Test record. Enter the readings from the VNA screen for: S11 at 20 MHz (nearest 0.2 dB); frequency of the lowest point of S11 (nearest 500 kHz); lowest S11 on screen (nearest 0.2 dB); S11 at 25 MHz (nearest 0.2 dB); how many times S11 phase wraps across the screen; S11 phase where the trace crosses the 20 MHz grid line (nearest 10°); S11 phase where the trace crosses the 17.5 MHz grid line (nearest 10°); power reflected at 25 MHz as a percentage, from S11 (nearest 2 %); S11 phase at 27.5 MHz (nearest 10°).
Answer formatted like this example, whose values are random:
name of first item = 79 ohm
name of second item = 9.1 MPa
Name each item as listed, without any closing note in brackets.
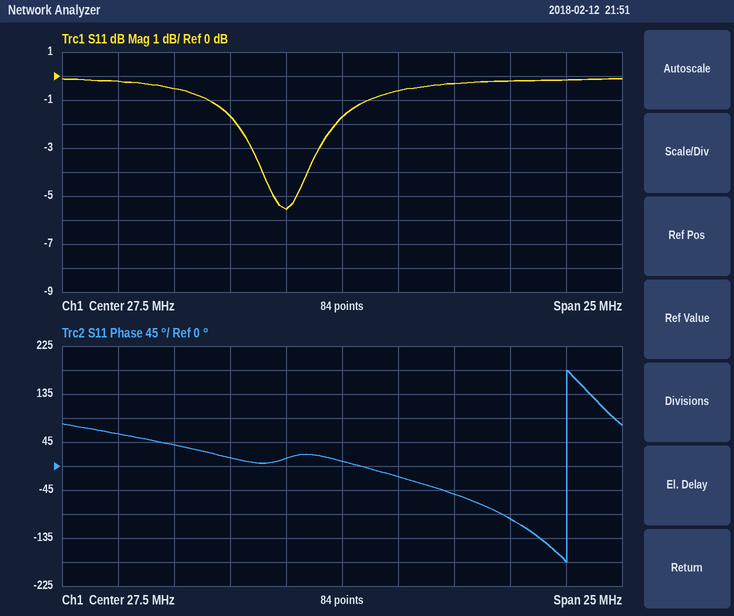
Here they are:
S11 at 20 MHz = -0.6 dB
frequency of the lowest point of S11 = 25.0 MHz
lowest S11 on screen = -5.6 dB
S11 at 25 MHz = -5.6 dB
how many times S11 phase wraps across the screen = 1
S11 phase where the trace crosses the 20 MHz grid line = 40°
S11 phase where the trace crosses the 17.5 MHz grid line = 60°
power reflected at 25 MHz as a percentage, from S11 = 28 %
S11 phase at 27.5 MHz = 10°
